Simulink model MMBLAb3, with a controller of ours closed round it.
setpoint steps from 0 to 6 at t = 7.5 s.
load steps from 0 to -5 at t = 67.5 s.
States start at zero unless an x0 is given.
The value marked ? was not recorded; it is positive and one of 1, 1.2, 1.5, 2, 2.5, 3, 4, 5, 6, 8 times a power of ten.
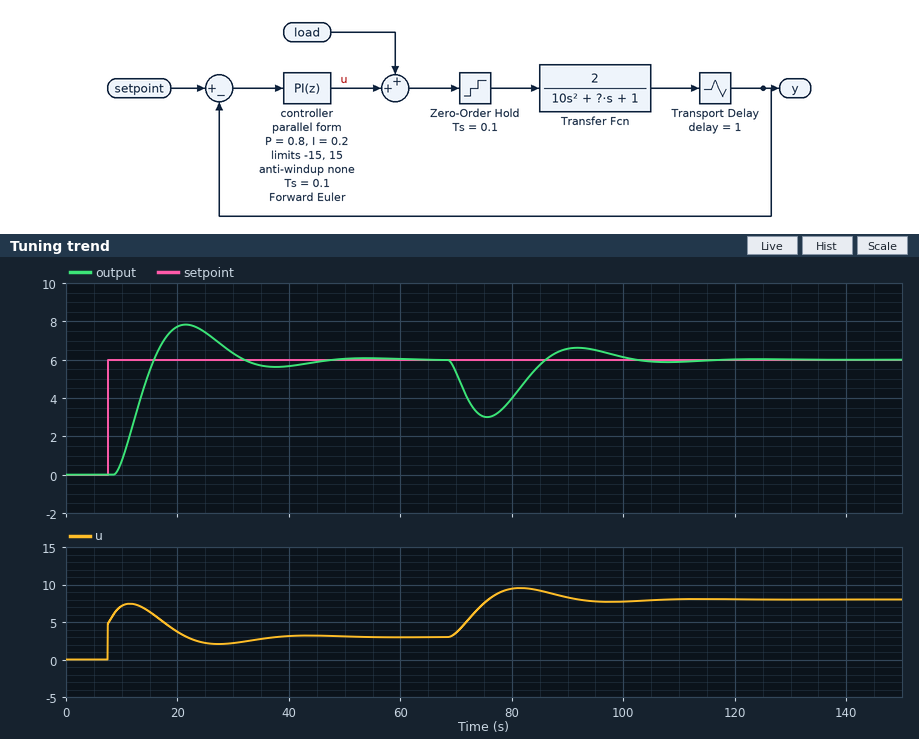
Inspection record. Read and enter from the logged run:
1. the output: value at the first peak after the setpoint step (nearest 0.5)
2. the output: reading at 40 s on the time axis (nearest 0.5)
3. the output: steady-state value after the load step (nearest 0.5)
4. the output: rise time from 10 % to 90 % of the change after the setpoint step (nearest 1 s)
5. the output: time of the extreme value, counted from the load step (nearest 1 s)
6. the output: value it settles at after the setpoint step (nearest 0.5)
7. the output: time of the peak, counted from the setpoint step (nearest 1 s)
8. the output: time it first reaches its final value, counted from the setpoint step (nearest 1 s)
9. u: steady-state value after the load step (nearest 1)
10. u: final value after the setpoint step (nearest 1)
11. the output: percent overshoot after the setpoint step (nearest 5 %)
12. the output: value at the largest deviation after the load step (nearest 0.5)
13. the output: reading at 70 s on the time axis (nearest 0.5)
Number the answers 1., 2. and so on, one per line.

1. 8.0
2. 5.5
3. 6.0
4. 5 s
5. 8 s
6. 6.0
7. 14 s
8. 8 s
9. 8
10. 3
11. 30 %
12. 3.0
13. 5.5
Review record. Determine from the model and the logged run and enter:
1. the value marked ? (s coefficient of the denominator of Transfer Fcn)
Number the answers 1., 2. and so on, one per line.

1. 12
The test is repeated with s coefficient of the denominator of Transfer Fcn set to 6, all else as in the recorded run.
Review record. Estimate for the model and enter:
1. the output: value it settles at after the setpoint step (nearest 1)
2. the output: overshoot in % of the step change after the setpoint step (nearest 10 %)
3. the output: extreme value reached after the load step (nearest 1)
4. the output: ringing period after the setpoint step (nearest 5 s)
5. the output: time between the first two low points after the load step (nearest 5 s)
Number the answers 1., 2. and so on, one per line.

1. 6
2. 40 %
3. 2
4. 15 s
5. 15 s
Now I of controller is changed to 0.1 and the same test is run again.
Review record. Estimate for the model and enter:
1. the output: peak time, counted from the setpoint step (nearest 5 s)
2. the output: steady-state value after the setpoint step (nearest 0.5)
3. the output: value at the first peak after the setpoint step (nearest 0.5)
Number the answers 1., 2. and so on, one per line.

1. 20 s
2. 6.0
3. 6.5
